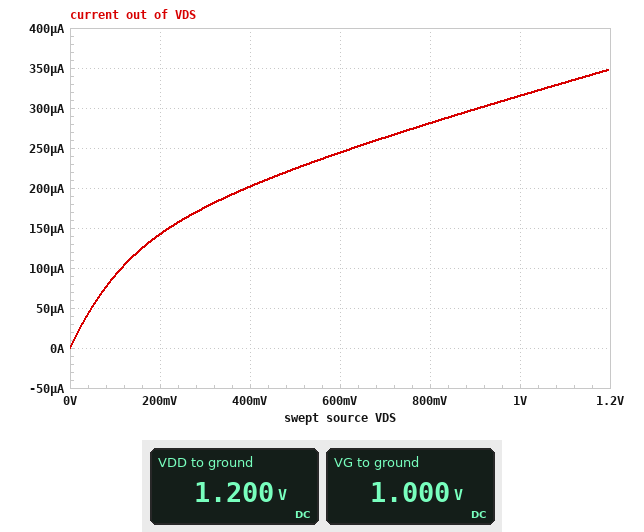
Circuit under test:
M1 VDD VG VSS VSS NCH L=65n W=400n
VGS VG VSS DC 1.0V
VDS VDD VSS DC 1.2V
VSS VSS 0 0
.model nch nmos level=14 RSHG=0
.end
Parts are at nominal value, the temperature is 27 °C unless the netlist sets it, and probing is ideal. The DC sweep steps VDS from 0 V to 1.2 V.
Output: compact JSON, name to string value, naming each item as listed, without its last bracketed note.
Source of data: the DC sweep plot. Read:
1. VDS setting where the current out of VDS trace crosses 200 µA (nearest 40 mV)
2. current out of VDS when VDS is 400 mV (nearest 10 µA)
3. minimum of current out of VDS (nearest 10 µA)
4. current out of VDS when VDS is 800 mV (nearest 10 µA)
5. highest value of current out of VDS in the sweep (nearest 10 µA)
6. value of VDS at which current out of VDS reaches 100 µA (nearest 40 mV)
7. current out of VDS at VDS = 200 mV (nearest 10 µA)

{"VDS setting where the current out of VDS trace crosses 200 µA": "400 mV", "current out of VDS when VDS is 400 mV": "200 µA", "minimum of current out of VDS": "0 A", "current out of VDS when VDS is 800 mV": "280 µA", "highest value of current out of VDS in the sweep": "350 µA", "value of VDS at which current out of VDS reaches 100 µA": "120 mV", "current out of VDS at VDS = 200 mV": "140 µA"}
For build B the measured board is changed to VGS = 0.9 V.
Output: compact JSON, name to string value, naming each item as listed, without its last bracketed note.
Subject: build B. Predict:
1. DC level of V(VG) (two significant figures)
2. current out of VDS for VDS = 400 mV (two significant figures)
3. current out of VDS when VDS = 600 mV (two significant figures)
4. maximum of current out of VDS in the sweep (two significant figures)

{"DC level of V(VG)": "900 mV", "current out of VDS for VDS = 400 mV": "170 µA", "current out of VDS when VDS = 600 mV": "210 µA", "maximum of current out of VDS in the sweep": "310 µA"}
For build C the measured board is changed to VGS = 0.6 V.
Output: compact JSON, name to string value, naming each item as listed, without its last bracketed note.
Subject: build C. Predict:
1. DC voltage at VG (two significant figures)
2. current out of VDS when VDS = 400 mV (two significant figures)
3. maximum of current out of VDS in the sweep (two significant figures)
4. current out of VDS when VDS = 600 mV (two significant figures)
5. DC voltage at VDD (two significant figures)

{"DC voltage at VG": "600 mV", "current out of VDS when VDS = 400 mV": "88 µA", "maximum of current out of VDS in the sweep": "190 µA", "current out of VDS when VDS = 600 mV": "110 µA", "DC voltage at VDD": "1.2 V"}
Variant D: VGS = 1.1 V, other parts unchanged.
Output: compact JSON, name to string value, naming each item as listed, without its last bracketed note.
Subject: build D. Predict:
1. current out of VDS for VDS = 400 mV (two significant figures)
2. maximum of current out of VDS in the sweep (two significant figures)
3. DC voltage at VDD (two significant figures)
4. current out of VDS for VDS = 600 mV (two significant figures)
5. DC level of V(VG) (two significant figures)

{"current out of VDS for VDS = 400 mV": "230 µA", "maximum of current out of VDS in the sweep": "390 µA", "DC voltage at VDD": "1.2 V", "current out of VDS for VDS = 600 mV": "280 µA", "DC level of V(VG)": "1.1 V"}
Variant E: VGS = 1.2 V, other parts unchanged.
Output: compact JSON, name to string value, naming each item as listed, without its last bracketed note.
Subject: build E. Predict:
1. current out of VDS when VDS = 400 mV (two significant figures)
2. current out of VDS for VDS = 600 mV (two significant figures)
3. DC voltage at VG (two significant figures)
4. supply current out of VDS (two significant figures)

{"current out of VDS when VDS = 400 mV": "260 µA", "current out of VDS for VDS = 600 mV": "310 µA", "DC voltage at VG": "1.2 V", "supply current out of VDS": "420 µA"}
